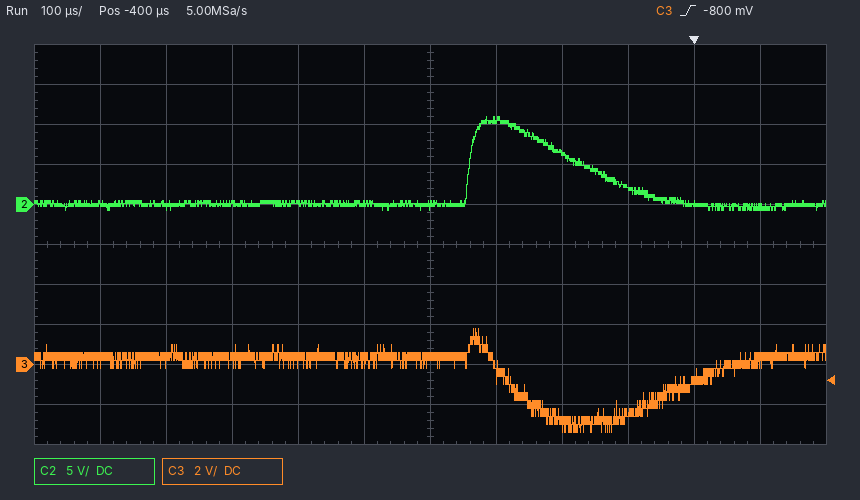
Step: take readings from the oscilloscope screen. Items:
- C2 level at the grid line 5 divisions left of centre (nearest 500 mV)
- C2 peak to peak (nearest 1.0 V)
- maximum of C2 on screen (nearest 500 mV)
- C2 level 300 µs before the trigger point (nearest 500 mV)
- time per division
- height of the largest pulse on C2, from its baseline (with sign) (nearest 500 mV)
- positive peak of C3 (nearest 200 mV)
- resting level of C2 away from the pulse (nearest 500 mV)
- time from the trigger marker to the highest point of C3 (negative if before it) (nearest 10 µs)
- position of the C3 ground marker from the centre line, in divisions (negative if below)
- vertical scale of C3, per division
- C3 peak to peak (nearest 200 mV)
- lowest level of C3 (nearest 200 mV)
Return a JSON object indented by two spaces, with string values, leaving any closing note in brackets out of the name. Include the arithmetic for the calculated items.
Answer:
{
  "C2 level at the grid line 5 divisions left of centre": "0.0 V",
  "C2 peak to peak": "12.0 V",
  "maximum of C2 on screen": "11.0 V",
  "C2 level 300 µs before the trigger point": "10.5 V",
  "time per division": "100 µs",
  "height of the largest pulse on C2, from its baseline (with sign)": "11.0 V − (0.0 V) = +11.0 V",
  "positive peak of C3": "1.8 V",
  "resting level of C2 away from the pulse": "0.0 V",
  "time from the trigger marker to the highest point of C3 (negative if before it)": "-330 µs",
  "position of the C3 ground marker from the centre line, in divisions": "-3.0 div",
  "vertical scale of C3, per division": "2 V",
  "C3 peak to peak": "1.8 V − (-3.4 V) = 5.2 V",
  "lowest level of C3": "-3.4 V"
}
